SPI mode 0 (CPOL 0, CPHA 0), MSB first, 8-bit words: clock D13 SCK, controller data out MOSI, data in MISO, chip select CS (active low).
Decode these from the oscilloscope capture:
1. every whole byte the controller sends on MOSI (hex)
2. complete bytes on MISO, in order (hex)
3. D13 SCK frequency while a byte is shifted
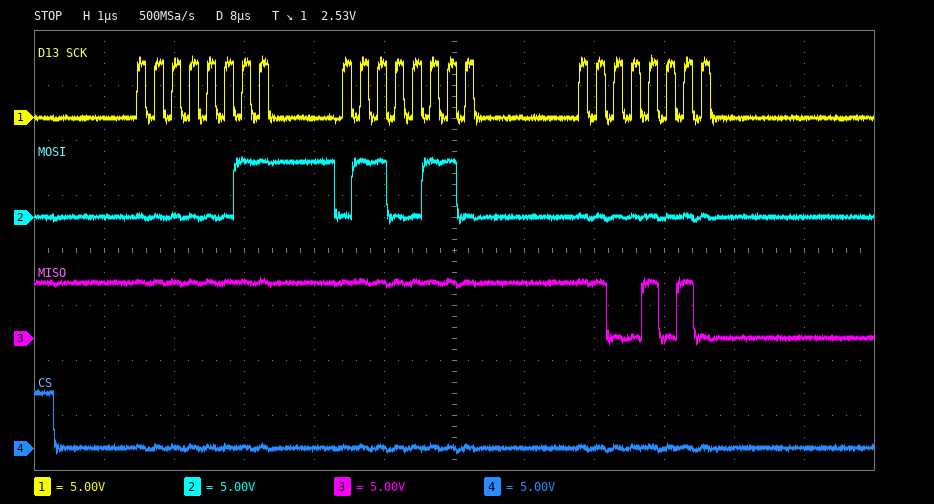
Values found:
0x03 0x66 0x00
0xFF 0xFF 0xCA
4 MHz
